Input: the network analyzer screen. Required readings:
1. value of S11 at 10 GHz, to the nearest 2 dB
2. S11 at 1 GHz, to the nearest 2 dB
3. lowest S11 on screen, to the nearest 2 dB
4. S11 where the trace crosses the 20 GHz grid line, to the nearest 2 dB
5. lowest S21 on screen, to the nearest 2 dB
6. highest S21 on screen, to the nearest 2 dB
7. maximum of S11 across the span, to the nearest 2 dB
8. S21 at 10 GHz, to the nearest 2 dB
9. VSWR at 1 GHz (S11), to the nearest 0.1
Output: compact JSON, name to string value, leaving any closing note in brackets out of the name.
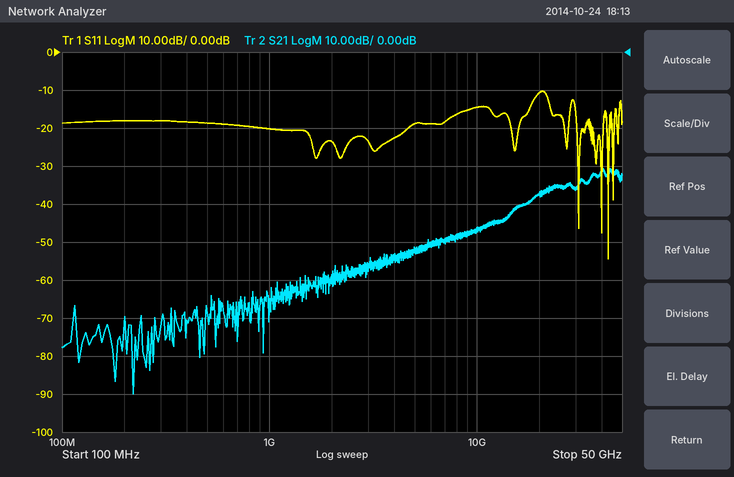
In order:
{"value of S11 at 10 GHz, to the nearest 2 dB": "-14 dB", "S11 at 1 GHz, to the nearest 2 dB": "-20 dB", "lowest S11 on screen, to the nearest 2 dB": "-54 dB", "S11 where the trace crosses the 20 GHz grid line, to the nearest 2 dB": "-10 dB", "lowest S21 on screen, to the nearest 2 dB": "-90 dB", "highest S21 on screen, to the nearest 2 dB": "-30 dB", "maximum of S11 across the span, to the nearest 2 dB": "-10 dB", "S21 at 10 GHz, to the nearest 2 dB": "-46 dB", "VSWR at 1 GHz (S11), to the nearest 0.1": "1.2"}
